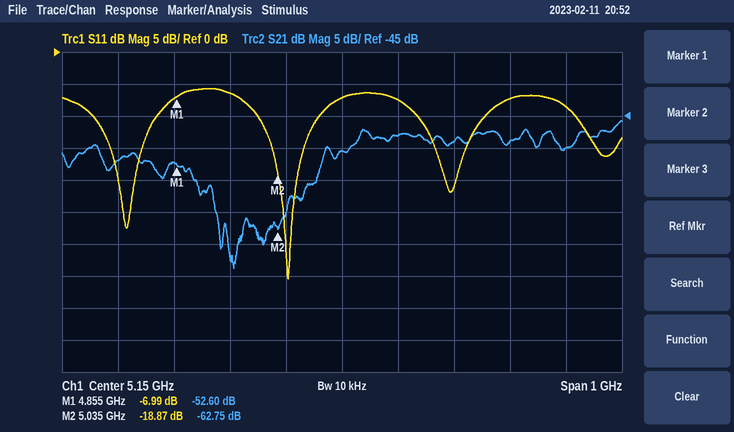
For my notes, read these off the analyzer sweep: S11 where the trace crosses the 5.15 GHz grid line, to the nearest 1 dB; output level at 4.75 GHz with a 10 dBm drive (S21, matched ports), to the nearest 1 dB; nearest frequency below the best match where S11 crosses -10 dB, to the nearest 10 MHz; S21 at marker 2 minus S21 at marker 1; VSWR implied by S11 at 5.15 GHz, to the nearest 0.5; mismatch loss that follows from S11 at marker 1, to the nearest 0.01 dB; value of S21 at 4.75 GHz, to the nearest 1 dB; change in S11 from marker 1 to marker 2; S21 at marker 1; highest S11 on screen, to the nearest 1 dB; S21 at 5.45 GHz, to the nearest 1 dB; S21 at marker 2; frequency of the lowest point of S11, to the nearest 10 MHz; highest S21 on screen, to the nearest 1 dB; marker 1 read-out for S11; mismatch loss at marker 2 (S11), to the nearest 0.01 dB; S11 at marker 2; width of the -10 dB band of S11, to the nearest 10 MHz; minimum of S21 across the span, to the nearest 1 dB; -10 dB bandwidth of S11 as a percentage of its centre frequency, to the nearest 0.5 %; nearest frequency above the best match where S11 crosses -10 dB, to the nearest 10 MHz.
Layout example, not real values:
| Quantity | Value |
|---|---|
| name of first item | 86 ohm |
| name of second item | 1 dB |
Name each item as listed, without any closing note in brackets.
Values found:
| Quantity | Value |
|---|---|
| S11 where the trace crosses the 5.15 GHz grid line, to the nearest 1 dB | -7 dB |
| output level at 4.75 GHz with a 10 dBm drive (S21, matched ports), to the nearest 1 dB | -42 dBm |
| nearest frequency below the best match where S11 crosses -10 dB, to the nearest 10 MHz | 5.00 GHz |
| S21 at marker 2 minus S21 at marker 1 | -10.15 dB |
| VSWR implied by S11 at 5.15 GHz, to the nearest 0.5 | 2.5 |
| mismatch loss that follows from S11 at marker 1, to the nearest 0.01 dB | 0.97 dB |
| value of S21 at 4.75 GHz, to the nearest 1 dB | -52 dB |
| change in S11 from marker 1 to marker 2 | -11.88 dB |
| S21 at marker 1 | -52.60 dB |
| highest S11 on screen, to the nearest 1 dB | -6 dB |
| S21 at 5.45 GHz, to the nearest 1 dB | -49 dB |
| S21 at marker 2 | -62.75 dB |
| frequency of the lowest point of S11, to the nearest 10 MHz | 5.05 GHz |
| highest S21 on screen, to the nearest 1 dB | -46 dB |
| marker 1 read-out for S11 | -6.99 dB |
| mismatch loss at marker 2 (S11), to the nearest 0.01 dB | 0.06 dB |
| S11 at marker 2 | -18.87 dB |
| width of the -10 dB band of S11, to the nearest 10 MHz | 110 MHz |
| minimum of S21 across the span, to the nearest 1 dB | -69 dB |
| -10 dB bandwidth of S11 as a percentage of its centre frequency, to the nearest 0.5 % | 2.0 % |
| nearest frequency above the best match where S11 crosses -10 dB, to the nearest 10 MHz | 5.11 GHz |
